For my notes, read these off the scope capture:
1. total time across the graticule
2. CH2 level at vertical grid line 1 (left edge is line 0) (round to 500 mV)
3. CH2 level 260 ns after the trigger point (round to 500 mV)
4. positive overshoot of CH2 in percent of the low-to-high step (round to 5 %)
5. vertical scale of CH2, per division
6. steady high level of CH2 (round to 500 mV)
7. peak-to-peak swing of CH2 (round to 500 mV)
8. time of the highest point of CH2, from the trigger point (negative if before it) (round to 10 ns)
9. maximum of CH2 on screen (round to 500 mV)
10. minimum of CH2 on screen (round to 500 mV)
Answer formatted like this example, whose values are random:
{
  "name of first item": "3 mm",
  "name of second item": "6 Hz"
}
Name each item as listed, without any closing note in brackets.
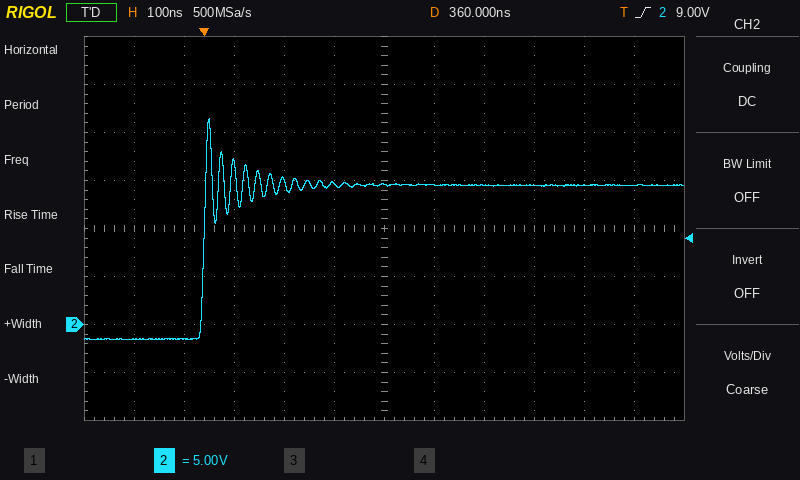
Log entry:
{
  "total time across the graticule": "1.2 µs",
  "CH2 level at vertical grid line 1 (left edge is line 0)": "-1.5 V",
  "CH2 level 260 ns after the trigger point": "14.5 V",
  "positive overshoot of CH2 in percent of the low-to-high step": "45 %",
  "vertical scale of CH2, per division": "5 V",
  "steady high level of CH2": "14.5 V",
  "peak-to-peak swing of CH2": "23.0 V",
  "time of the highest point of CH2, from the trigger point (negative if before it)": "+10 ns",
  "maximum of CH2 on screen": "21.5 V",
  "minimum of CH2 on screen": "-1.5 V"
}
